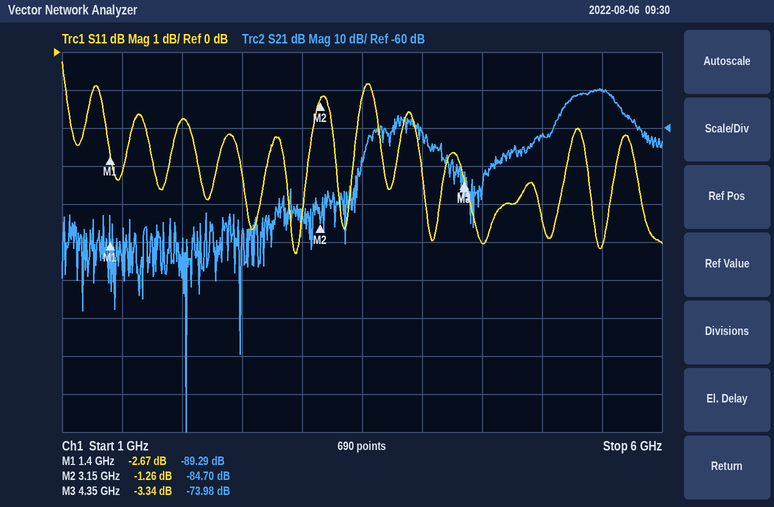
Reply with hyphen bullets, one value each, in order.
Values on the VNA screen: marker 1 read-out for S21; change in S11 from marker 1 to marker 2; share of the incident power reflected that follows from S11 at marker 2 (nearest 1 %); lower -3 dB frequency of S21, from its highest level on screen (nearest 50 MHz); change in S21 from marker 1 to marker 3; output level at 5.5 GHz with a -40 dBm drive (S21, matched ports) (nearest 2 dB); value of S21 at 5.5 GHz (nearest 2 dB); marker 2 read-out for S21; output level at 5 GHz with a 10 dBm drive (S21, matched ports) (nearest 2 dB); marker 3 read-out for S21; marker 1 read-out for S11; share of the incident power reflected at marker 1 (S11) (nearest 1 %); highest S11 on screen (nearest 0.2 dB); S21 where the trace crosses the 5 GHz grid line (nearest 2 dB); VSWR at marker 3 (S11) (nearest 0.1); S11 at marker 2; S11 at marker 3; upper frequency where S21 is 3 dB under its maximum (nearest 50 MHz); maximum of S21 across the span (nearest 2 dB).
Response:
- -89.29 dB
- 1.41 dB
- 75 %
- 5.25 GHz
- 15.31 dB
- -90 dBm
- -50 dB
- -84.70 dB
- -52 dBm
- -73.98 dB
- -2.67 dB
- 54 %
- -0.2 dB
- -62 dB
- 5.3
- -1.26 dB
- -3.34 dB
- 5.60 GHz
- -50 dB
